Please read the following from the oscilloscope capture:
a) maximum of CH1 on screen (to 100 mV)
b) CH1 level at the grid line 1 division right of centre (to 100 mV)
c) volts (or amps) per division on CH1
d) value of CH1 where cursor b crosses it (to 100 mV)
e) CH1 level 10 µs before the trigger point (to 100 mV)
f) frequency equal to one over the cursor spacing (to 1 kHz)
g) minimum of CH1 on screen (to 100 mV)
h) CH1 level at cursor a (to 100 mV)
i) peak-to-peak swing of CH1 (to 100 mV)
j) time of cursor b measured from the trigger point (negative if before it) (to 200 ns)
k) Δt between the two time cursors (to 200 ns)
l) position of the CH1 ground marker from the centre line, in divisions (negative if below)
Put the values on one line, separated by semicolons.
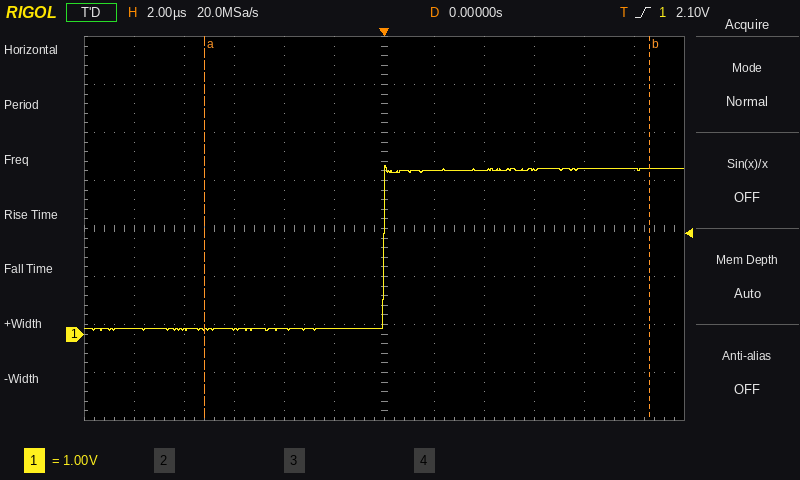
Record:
3.5 V; 3.4 V; 1 V; 3.4 V; 100 mV; 56 kHz; 100 mV; 100 mV; 3.4 V; +10.6 µs; 17.8 µs; -2.2 div
